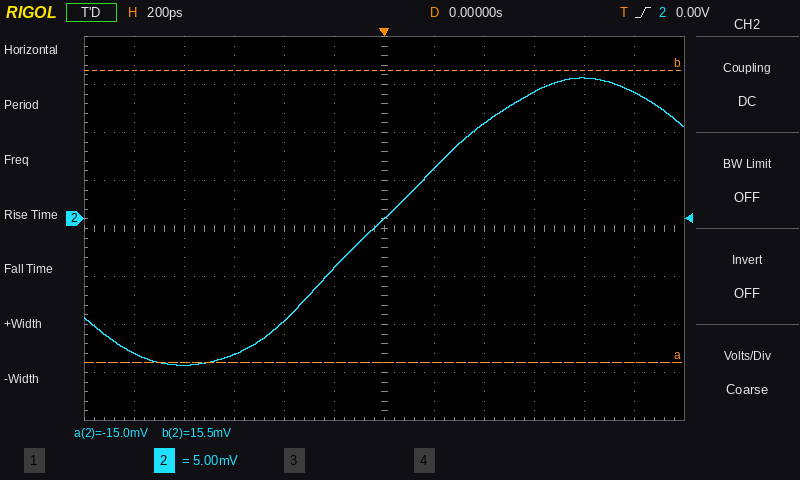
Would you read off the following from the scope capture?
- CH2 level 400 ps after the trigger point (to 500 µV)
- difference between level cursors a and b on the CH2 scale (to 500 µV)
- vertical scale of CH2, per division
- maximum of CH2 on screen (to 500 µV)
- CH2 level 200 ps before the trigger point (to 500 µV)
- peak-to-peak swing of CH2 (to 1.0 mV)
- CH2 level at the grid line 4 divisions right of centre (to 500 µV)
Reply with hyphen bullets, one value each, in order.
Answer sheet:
- 10.0 mV
- 30.5 mV
- 5 mV
- 14.5 mV
- -5.0 mV
- 30.0 mV
- 14.5 mV
